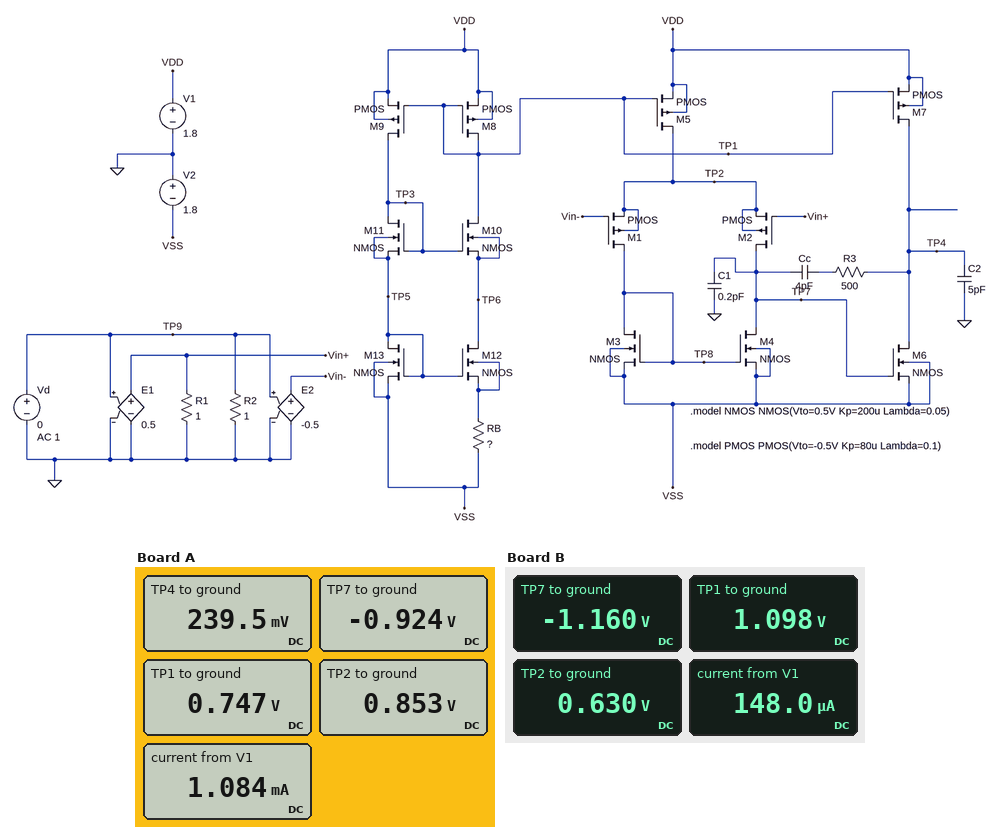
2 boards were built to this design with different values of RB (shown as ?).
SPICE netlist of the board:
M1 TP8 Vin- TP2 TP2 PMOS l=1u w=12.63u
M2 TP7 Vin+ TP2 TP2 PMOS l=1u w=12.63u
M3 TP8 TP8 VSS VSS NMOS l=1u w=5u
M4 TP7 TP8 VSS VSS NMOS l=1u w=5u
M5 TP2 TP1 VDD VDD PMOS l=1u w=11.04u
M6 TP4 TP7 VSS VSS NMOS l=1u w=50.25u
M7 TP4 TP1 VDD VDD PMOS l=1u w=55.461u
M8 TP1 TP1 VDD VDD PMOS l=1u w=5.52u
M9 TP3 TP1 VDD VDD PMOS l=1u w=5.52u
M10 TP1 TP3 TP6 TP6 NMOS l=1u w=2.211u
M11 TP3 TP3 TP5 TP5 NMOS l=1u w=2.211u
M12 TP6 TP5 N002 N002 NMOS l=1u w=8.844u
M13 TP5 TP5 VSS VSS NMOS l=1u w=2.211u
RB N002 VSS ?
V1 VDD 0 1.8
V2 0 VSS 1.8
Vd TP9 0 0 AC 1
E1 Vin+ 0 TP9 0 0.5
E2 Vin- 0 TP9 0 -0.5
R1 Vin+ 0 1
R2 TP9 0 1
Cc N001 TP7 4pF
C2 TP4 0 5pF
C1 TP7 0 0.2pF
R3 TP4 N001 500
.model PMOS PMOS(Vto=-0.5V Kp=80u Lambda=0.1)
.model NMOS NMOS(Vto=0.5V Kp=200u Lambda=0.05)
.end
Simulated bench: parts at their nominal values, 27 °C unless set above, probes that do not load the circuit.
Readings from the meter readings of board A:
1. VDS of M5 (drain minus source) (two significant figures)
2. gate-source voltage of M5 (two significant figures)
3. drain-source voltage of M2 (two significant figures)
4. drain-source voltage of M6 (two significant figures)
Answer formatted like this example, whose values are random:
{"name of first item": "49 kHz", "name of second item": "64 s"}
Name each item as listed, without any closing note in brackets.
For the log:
{"VDS of M5 (drain minus source)": "-950 mV", "gate-source voltage of M5": "-1.1 V", "drain-source voltage of M2": "-1.8 V", "drain-source voltage of M6": "2.0 V"}
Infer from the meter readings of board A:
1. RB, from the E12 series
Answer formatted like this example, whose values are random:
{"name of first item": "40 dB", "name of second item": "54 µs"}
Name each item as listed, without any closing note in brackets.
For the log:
{"RB, from the E12 series": "3.9 kΩ"}
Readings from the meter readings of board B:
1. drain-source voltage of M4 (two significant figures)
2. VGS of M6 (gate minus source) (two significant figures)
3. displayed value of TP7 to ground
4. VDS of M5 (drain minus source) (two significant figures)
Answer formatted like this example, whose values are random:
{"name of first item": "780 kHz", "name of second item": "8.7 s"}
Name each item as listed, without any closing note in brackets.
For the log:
{"drain-source voltage of M4": "640 mV", "VGS of M6 (gate minus source)": "640 mV", "displayed value of TP7 to ground": "-1.160 V", "VDS of M5 (drain minus source)": "-1.2 V"}
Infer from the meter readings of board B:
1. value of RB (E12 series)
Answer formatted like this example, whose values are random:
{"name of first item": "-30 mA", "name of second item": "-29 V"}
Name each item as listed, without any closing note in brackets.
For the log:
{"value of RB": "12 kΩ"}
